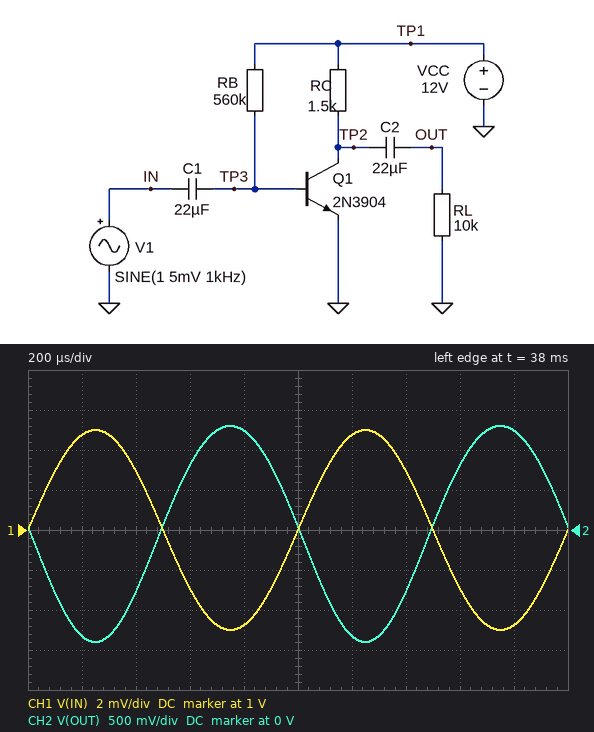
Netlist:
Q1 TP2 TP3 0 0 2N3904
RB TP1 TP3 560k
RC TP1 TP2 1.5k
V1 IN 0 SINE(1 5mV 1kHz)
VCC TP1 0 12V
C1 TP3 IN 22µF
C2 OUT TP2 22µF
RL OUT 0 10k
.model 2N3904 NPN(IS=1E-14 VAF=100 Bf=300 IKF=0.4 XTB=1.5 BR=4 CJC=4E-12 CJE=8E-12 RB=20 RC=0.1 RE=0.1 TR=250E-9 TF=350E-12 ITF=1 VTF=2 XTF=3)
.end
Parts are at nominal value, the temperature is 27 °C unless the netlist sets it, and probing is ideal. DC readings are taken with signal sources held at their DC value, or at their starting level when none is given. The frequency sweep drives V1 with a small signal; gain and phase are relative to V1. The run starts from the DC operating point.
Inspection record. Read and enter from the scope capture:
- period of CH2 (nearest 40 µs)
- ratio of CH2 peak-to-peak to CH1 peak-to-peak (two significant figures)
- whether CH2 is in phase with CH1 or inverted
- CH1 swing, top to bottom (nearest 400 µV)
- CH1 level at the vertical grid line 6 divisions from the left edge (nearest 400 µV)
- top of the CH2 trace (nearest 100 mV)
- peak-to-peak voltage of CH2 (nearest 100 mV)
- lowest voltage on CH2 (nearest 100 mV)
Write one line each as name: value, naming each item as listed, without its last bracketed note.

period of CH2: 1.00 ms
ratio of CH2 peak-to-peak to CH1 peak-to-peak: 270
whether CH2 is in phase with CH1 or inverted: inverted
CH1 swing, top to bottom: 10.0 mV
CH1 level at the vertical grid line 6 divisions from the left edge: 1.0048 V
top of the CH2 trace: 1.3 V
peak-to-peak voltage of CH2: 2.7 V
lowest voltage on CH2: -1.4 V
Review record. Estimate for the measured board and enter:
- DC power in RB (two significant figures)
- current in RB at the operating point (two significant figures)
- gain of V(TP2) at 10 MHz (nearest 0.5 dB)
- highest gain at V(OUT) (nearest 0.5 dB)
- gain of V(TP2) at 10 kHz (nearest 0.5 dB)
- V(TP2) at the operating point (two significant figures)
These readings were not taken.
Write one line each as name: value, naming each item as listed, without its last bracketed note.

DC power in RB: 230 µW
current in RB at the operating point: 20 µA
gain of V(TP2) at 10 MHz: 45.0 dB
highest gain at V(OUT): 48.5 dB
gain of V(TP2) at 10 kHz: 48.5 dB
V(TP2) at the operating point: 2.9 V
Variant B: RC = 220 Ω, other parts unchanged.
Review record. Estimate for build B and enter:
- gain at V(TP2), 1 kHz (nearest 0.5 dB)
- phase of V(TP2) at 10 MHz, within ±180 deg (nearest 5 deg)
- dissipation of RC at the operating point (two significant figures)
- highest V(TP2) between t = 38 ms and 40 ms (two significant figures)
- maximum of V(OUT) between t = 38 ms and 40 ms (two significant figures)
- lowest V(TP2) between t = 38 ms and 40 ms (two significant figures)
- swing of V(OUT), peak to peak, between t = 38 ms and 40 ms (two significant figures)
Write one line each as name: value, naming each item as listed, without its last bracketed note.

gain at V(TP2), 1 kHz: 34.0 dB
phase of V(TP2) at 10 MHz, within ±180 deg: 165 deg
dissipation of RC at the operating point: 9.4 mW
highest V(TP2) between t = 38 ms and 40 ms: 11 V
maximum of V(OUT) between t = 38 ms and 40 ms: 240 mV
lowest V(TP2) between t = 38 ms and 40 ms: 10 V
swing of V(OUT), peak to peak, between t = 38 ms and 40 ms: 510 mV
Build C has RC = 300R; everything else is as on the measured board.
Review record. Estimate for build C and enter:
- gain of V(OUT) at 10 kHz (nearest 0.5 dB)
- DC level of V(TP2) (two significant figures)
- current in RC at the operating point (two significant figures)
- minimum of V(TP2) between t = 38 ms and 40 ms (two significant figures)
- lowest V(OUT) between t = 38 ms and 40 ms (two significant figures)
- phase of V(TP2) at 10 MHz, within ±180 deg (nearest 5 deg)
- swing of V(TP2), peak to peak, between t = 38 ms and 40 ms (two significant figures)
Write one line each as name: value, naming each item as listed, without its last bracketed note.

gain of V(OUT) at 10 kHz: 36.5 dB
DC level of V(TP2): 10 V
current in RC at the operating point: 6.5 mA
minimum of V(TP2) between t = 38 ms and 40 ms: 9.7 V
lowest V(OUT) between t = 38 ms and 40 ms: -360 mV
phase of V(TP2) at 10 MHz, within ±180 deg: 165 deg
swing of V(TP2), peak to peak, between t = 38 ms and 40 ms: 680 mV
